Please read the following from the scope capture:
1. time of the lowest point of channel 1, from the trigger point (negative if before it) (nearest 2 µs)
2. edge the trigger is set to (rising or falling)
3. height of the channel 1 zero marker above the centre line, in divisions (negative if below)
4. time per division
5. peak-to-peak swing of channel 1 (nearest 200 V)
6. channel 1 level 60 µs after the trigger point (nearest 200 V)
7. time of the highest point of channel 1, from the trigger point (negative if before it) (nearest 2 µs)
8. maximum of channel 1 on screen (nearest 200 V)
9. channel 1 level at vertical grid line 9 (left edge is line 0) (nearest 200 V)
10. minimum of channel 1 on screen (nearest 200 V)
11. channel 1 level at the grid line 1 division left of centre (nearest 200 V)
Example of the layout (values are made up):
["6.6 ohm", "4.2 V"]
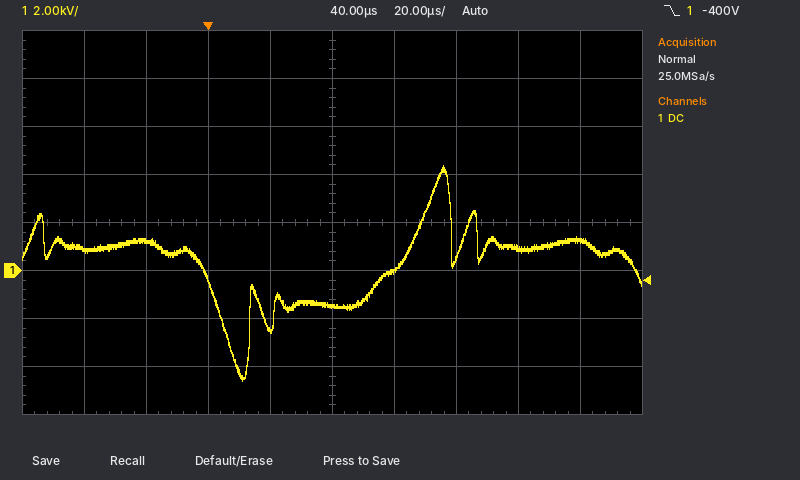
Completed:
["+12 µs", "falling", "-1.0 div", "20 µs", "9.0 kV", "0.0 kV", "+76 µs", "4.4 kV", "1.2 kV", "-4.6 kV", "-2.4 kV"]
